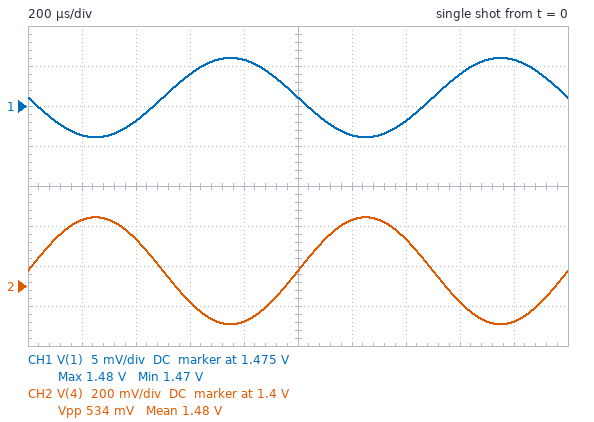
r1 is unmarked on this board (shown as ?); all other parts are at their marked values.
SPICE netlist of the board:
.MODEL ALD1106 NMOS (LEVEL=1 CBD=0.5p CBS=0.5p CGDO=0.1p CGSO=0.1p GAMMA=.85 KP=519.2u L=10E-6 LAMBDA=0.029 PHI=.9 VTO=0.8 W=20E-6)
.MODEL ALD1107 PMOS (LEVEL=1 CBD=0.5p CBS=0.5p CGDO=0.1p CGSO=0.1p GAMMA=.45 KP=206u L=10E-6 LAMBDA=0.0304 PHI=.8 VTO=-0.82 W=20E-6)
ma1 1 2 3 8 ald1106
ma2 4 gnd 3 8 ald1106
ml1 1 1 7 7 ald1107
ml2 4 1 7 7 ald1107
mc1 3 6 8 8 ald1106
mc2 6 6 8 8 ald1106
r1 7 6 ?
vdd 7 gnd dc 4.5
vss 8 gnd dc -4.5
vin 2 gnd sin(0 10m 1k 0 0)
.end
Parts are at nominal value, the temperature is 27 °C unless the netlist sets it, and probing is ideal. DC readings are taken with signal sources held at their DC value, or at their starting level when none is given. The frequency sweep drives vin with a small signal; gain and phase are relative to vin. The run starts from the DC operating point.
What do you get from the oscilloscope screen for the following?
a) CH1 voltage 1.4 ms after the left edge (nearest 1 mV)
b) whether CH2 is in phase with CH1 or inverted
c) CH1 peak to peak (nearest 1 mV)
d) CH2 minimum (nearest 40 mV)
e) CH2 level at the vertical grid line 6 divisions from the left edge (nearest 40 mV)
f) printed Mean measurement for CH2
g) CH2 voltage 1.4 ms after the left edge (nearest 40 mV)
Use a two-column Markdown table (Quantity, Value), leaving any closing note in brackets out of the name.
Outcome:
| Quantity | Value |
|---|---|
| CH1 voltage 1.4 ms after the left edge | 1.473 V |
| whether CH2 is in phase with CH1 or inverted | inverted |
| CH1 peak to peak | 10 mV |
| CH2 minimum | 1.20 V |
| CH2 level at the vertical grid line 6 divisions from the left edge | 1.72 V |
| printed Mean measurement for CH2 | 1.48 V |
| CH2 voltage 1.4 ms after the left edge | 1.64 V |
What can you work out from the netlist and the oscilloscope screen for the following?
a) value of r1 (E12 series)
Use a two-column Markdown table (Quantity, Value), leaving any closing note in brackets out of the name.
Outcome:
| Quantity | Value |
|---|---|
| value of r1 | 2.7 kΩ |
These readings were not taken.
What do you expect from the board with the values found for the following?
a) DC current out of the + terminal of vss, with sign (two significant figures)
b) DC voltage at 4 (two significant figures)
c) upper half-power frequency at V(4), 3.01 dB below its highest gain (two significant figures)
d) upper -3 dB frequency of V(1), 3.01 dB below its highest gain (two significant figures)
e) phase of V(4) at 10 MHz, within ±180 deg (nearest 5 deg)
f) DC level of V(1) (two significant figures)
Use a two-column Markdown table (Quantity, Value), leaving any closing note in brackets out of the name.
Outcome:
| Quantity | Value |
|---|---|
| DC current out of the + terminal of vss, with sign | -4.5 mA |
| DC voltage at 4 | 1.5 V |
| upper half-power frequency at V(4), 3.01 dB below its highest gain | 23 MHz |
| upper -3 dB frequency of V(1), 3.01 dB below its highest gain | 720 MHz |
| phase of V(4) at 10 MHz, within ±180 deg | -25 deg |
| DC level of V(1) | 1.5 V |
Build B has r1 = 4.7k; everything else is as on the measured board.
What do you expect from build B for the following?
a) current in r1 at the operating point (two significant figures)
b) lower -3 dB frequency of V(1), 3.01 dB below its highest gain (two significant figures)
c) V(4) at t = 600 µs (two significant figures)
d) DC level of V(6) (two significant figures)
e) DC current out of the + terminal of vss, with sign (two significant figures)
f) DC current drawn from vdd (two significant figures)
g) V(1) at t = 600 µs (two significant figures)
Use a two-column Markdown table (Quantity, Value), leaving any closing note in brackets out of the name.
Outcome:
| Quantity | Value |
|---|---|
| current in r1 at the operating point | 1.4 mA |
| lower -3 dB frequency of V(1), 3.01 dB below its highest gain | 9.1 MHz |
| V(4) at t = 600 µs | 1.7 V |
| DC level of V(6) | -2.1 V |
| DC current out of the + terminal of vss, with sign | -2.8 mA |
| DC current drawn from vdd | 2.8 mA |
| V(1) at t = 600 µs | 1.9 V |
